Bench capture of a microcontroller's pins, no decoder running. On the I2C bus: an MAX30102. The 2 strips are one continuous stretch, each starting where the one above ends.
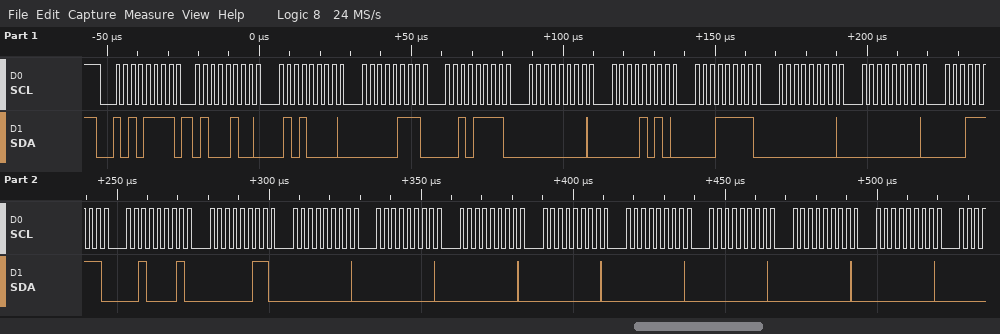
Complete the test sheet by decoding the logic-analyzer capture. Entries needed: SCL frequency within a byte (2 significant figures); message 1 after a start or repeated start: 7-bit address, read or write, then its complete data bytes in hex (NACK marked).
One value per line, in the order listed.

400 kHz
0x57 read: 44 50 07 2F 00 0A 1F 00 00 1F 21 03 00 00 00 00 00 00 00 00
